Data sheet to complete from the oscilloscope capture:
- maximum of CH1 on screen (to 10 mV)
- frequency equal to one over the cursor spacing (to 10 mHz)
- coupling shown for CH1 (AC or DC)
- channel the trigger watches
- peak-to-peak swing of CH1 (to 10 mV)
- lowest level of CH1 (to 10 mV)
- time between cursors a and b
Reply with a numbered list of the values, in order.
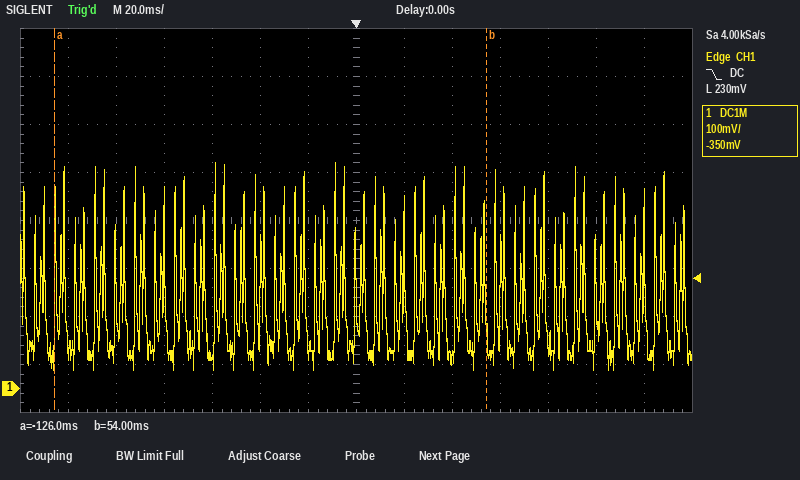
1. 470 mV
2. 5.56 Hz
3. DC
4. CH1
5. 430 mV
6. 40 mV
7. 180 ms
